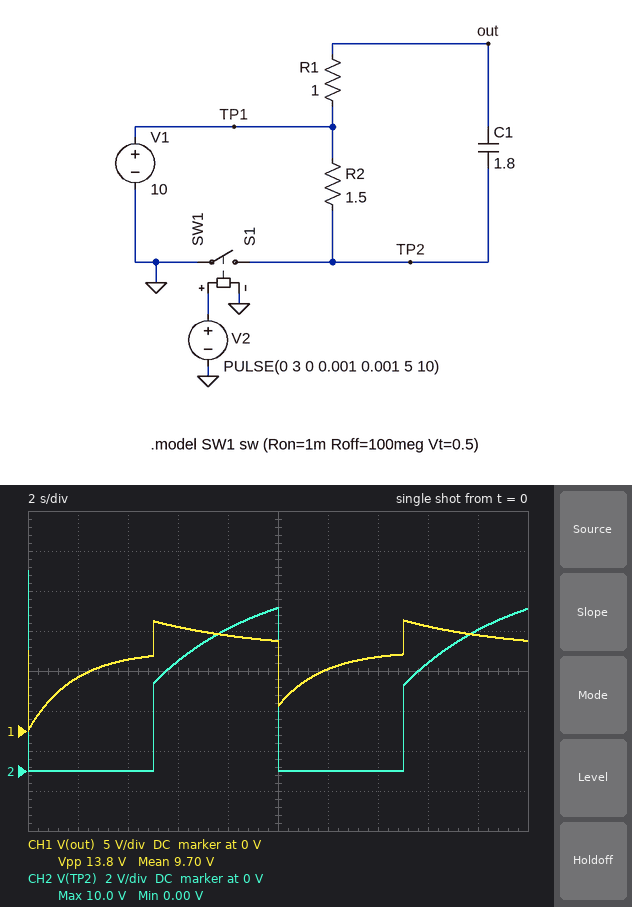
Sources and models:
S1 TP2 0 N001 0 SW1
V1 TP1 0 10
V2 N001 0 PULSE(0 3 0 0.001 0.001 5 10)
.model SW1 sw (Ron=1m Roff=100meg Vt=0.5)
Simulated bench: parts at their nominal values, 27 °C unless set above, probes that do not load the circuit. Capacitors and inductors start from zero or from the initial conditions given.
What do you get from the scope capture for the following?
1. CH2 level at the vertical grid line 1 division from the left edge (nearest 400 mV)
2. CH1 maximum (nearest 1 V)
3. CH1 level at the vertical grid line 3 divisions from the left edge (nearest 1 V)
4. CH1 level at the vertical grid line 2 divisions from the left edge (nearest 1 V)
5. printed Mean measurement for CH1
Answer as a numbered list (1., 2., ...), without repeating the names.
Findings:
1. 0 V
2. 14 V
3. 13 V
4. 9 V
5. 9.70 V
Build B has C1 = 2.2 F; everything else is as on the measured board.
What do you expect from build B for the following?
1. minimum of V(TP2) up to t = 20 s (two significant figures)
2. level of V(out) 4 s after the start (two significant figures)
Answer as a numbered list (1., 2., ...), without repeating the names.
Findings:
1. 7.3 mV
2. 8.4 V
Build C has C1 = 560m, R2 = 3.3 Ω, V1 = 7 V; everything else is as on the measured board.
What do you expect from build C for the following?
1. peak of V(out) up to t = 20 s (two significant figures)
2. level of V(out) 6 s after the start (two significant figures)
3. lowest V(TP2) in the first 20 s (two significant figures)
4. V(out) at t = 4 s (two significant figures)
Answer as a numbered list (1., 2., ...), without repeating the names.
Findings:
1. 8.6 V
2. 8.1 V
3. 2.1 mV
4. 7.0 V
